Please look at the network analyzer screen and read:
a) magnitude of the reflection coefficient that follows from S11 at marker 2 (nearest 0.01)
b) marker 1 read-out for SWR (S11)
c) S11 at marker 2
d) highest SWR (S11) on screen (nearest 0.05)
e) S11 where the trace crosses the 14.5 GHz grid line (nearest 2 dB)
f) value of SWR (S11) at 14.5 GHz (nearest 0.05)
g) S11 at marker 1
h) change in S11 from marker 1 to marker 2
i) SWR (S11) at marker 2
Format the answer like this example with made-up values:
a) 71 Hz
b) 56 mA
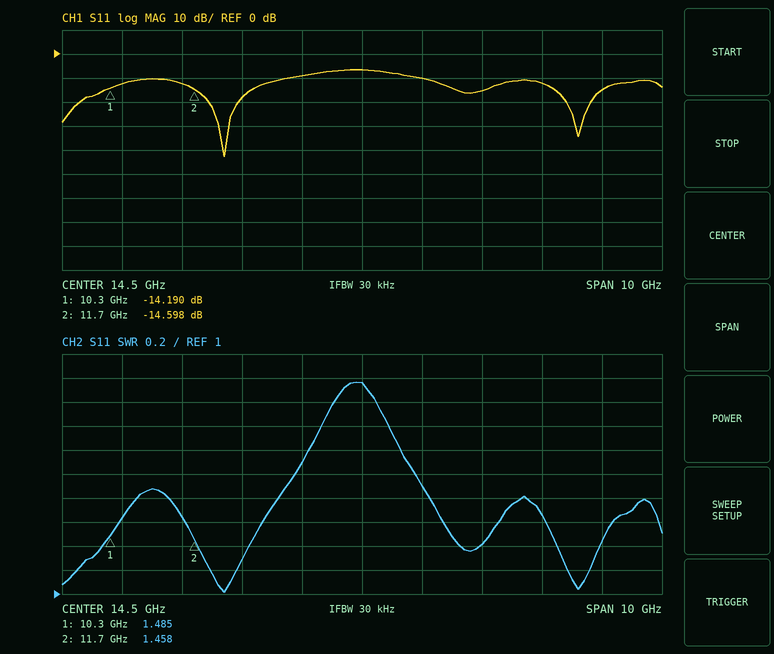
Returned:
a) 0.19
b) 1.485
c) -14.598 dB
d) 2.75
e) -6 dB
f) 2.75
g) -14.190 dB
h) -0.408 dB
i) 1.458
